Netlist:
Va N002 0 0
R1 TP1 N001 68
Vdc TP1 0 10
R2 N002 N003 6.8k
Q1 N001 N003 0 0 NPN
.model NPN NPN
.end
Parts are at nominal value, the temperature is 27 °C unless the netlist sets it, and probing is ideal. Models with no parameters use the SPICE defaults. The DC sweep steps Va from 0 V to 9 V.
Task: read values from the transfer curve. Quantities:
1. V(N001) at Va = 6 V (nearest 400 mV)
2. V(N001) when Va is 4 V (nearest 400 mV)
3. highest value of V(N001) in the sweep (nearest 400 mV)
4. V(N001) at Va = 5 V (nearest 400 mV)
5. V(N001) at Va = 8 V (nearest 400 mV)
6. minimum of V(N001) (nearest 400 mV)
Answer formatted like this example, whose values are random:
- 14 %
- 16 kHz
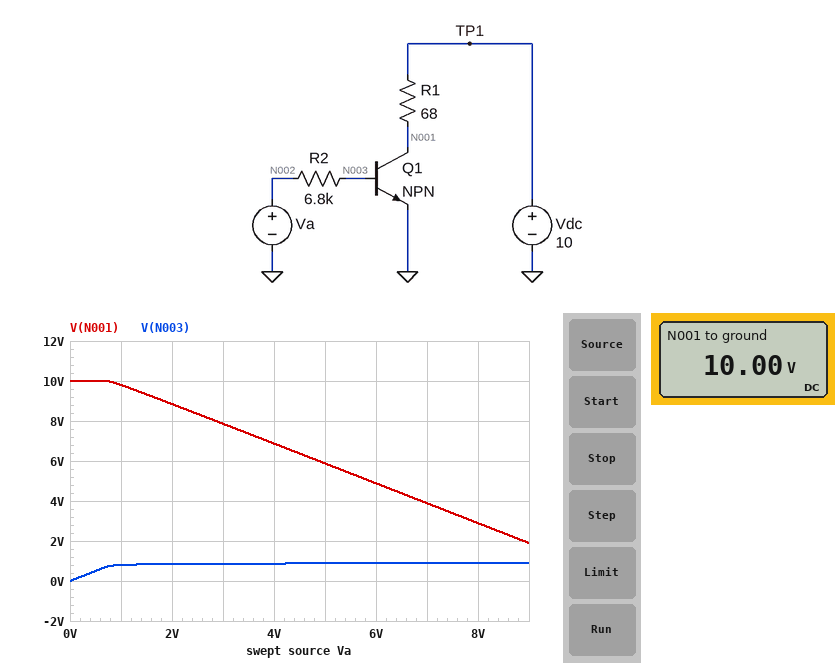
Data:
- 4.8 V
- 6.8 V
- 10.0 V
- 6.0 V
- 2.8 V
- 2.0 V
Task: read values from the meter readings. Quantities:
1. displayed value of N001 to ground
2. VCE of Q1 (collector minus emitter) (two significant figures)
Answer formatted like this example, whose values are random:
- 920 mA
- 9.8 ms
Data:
- 10.00 V
- 10 V
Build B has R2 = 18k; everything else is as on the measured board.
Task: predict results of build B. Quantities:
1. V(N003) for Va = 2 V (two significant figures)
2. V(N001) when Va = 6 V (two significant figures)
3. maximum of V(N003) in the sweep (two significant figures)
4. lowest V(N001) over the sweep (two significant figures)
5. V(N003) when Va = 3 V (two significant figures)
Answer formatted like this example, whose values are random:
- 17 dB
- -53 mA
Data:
- 820 mV
- 8.1 V
- 870 mV
- 6.9 V
- 840 mV
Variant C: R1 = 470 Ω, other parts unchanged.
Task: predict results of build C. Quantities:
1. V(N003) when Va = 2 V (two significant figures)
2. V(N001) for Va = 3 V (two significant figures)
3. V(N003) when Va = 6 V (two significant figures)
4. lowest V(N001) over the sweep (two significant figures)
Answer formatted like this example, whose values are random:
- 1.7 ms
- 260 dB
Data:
- 850 mV
- 140 mV
- 850 mV
- 82 mV
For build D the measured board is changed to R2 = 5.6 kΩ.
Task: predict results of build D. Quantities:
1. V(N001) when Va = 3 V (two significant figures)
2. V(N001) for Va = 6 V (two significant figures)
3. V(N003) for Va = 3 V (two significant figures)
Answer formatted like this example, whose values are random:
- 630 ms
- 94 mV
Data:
- 7.4 V
- 3.8 V
- 870 mV
